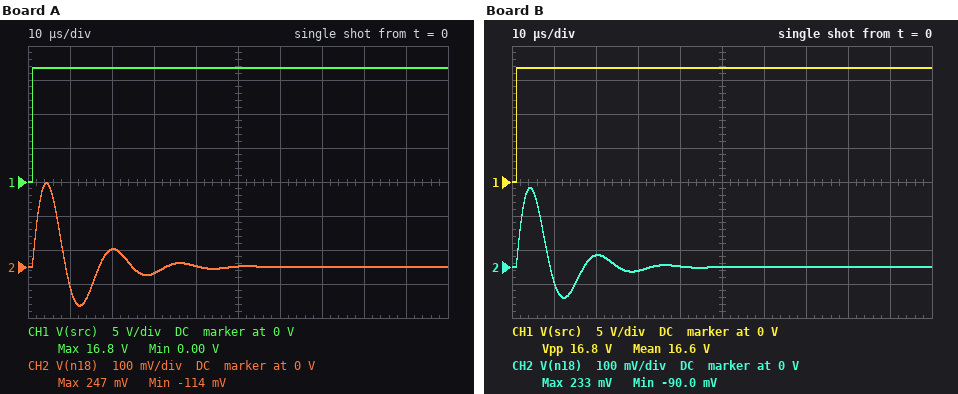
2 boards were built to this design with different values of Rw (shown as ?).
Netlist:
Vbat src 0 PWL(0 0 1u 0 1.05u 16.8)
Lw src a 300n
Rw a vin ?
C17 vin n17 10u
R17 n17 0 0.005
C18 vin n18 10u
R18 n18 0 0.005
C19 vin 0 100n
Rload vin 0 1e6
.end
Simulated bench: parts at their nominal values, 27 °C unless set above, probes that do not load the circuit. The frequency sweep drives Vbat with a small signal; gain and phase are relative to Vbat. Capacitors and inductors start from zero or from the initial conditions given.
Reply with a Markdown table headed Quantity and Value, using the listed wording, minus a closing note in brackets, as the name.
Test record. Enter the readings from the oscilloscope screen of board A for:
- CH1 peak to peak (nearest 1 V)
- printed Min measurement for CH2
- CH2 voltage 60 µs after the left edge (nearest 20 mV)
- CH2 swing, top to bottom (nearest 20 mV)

| Quantity | Value |
|---|---|
| CH1 peak to peak | 17 V |
| printed Min measurement for CH2 | -114 mV |
| CH2 voltage 60 µs after the left edge | 0 V |
| CH2 swing, top to bottom | 360 mV |
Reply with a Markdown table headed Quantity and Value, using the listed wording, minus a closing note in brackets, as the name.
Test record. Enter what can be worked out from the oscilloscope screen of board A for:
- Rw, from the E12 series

| Quantity | Value |
|---|---|
| Rw, from the E12 series | 0.056 Ω |
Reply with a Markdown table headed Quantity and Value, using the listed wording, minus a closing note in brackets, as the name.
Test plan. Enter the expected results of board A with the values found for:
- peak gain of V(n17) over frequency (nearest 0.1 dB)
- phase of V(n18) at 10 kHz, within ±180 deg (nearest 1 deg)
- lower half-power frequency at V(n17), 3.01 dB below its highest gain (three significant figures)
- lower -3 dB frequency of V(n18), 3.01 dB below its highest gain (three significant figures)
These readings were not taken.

| Quantity | Value |
|---|---|
| peak gain of V(n17) over frequency | -27.4 dB |
| phase of V(n18) at 10 kHz, within ±180 deg | 86 deg |
| lower half-power frequency at V(n17), 3.01 dB below its highest gain | 51.1 kHz |
| lower -3 dB frequency of V(n18), 3.01 dB below its highest gain | 51.1 kHz |
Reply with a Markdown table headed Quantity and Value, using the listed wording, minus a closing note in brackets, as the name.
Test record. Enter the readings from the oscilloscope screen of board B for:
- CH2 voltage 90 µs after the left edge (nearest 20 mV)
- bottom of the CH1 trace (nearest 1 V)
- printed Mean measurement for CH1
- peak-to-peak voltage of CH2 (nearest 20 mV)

| Quantity | Value |
|---|---|
| CH2 voltage 90 µs after the left edge | 0 V |
| bottom of the CH1 trace | 0 V |
| printed Mean measurement for CH1 | 16.6 V |
| peak-to-peak voltage of CH2 | 320 mV |
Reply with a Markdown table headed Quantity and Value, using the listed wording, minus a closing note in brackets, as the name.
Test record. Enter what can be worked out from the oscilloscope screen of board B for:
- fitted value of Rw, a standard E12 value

| Quantity | Value |
|---|---|
| fitted value of Rw, a standard E12 value | 0.068 Ω |
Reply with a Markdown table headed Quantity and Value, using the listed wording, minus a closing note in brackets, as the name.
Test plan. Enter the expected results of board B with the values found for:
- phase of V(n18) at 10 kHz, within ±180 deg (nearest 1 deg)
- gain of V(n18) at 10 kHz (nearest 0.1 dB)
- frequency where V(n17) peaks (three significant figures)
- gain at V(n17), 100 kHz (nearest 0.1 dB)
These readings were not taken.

| Quantity | Value |
|---|---|
| phase of V(n18) at 10 kHz, within ±180 deg | 85 deg |
| gain of V(n18) at 10 kHz | -49.9 dB |
| frequency where V(n17) peaks | 64.8 kHz |
| gain at V(n17), 100 kHz | -34.4 dB |
